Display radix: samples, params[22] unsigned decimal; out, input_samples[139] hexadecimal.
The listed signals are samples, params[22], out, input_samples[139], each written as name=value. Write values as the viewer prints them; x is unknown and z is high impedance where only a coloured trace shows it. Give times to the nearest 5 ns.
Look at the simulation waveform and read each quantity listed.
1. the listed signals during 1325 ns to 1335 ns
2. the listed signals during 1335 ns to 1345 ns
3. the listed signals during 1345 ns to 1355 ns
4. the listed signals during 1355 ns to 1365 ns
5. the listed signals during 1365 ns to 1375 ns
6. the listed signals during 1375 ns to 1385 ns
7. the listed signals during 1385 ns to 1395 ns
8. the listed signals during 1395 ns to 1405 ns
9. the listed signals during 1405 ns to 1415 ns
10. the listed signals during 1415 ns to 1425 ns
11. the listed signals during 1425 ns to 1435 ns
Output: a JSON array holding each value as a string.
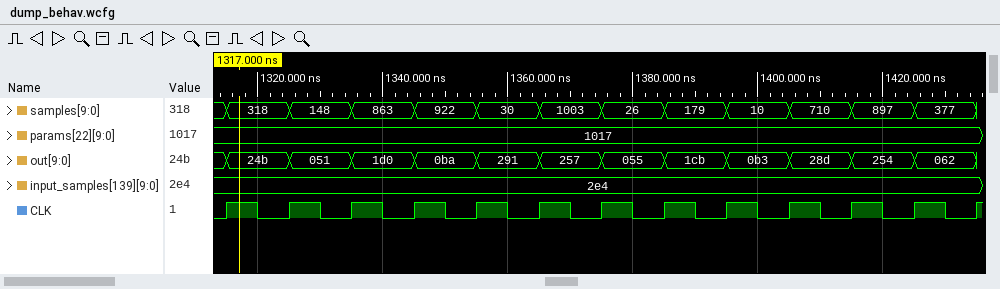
["samples=148, params[22]=1017, out=051, input_samples[139]=2e4", "samples=863, params[22]=1017, out=1d0, input_samples[139]=2e4", "samples=922, params[22]=1017, out=0ba, input_samples[139]=2e4", "samples=30, params[22]=1017, out=291, input_samples[139]=2e4", "samples=1003, params[22]=1017, out=257, input_samples[139]=2e4", "samples=26, params[22]=1017, out=055, input_samples[139]=2e4", "samples=179, params[22]=1017, out=1cb, input_samples[139]=2e4", "samples=10, params[22]=1017, out=0b3, input_samples[139]=2e4", "samples=710, params[22]=1017, out=28d, input_samples[139]=2e4", "samples=897, params[22]=1017, out=254, input_samples[139]=2e4", "samples=377, params[22]=1017, out=062, input_samples[139]=2e4"]
